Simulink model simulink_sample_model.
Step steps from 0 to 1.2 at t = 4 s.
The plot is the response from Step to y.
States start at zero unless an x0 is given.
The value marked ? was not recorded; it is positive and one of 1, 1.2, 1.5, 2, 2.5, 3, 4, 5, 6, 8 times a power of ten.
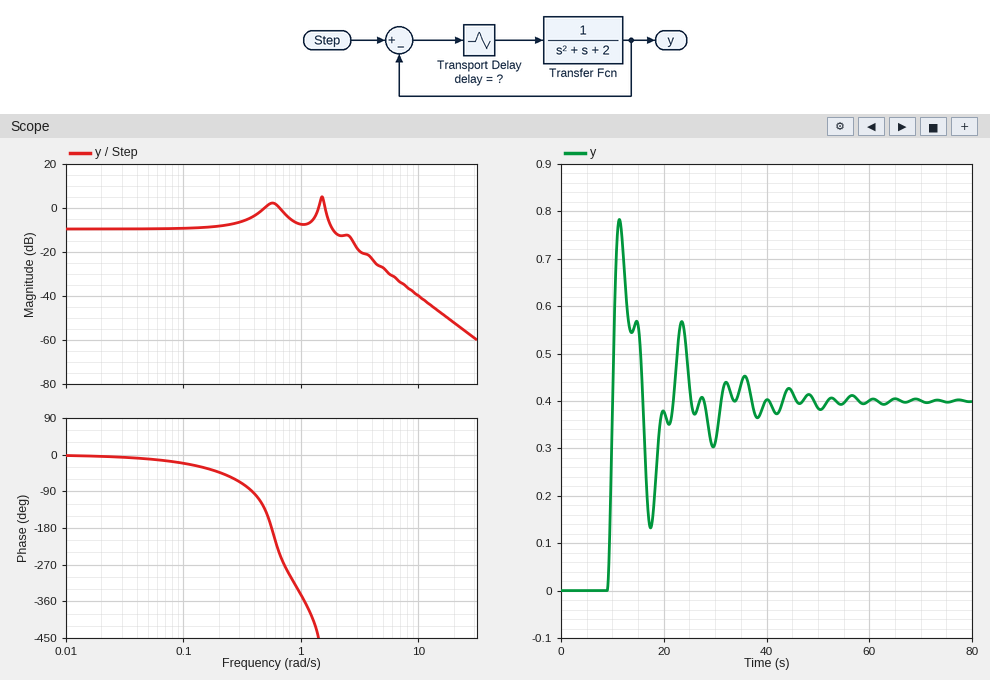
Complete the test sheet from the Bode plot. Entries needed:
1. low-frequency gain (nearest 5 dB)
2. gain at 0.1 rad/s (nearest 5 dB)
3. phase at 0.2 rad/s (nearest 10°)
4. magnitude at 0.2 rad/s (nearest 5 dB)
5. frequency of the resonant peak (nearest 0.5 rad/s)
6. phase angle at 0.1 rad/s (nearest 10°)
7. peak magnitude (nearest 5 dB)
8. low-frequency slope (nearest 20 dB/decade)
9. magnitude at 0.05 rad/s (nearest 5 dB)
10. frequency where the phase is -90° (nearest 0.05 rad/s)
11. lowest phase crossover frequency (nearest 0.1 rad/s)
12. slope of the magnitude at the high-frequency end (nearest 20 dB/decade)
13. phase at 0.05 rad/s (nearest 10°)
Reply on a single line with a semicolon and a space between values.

-10 dB; -10 dB; -40°; -10 dB; 1.5 rad/s; -20°; 5 dB; 0 dB/decade; -10 dB; 0.40 rad/s; 0.6 rad/s; -40 dB/decade; -10°
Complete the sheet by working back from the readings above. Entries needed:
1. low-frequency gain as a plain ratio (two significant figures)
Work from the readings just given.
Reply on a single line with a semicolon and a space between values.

0.32
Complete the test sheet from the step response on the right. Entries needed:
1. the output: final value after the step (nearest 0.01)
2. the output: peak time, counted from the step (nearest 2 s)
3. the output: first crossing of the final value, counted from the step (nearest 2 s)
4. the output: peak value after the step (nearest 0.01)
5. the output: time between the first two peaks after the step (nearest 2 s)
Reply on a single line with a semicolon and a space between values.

0.40; 8 s; 6 s; 0.78; 12 s
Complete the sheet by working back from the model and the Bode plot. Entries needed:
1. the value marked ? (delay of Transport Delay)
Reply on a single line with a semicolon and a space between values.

5
